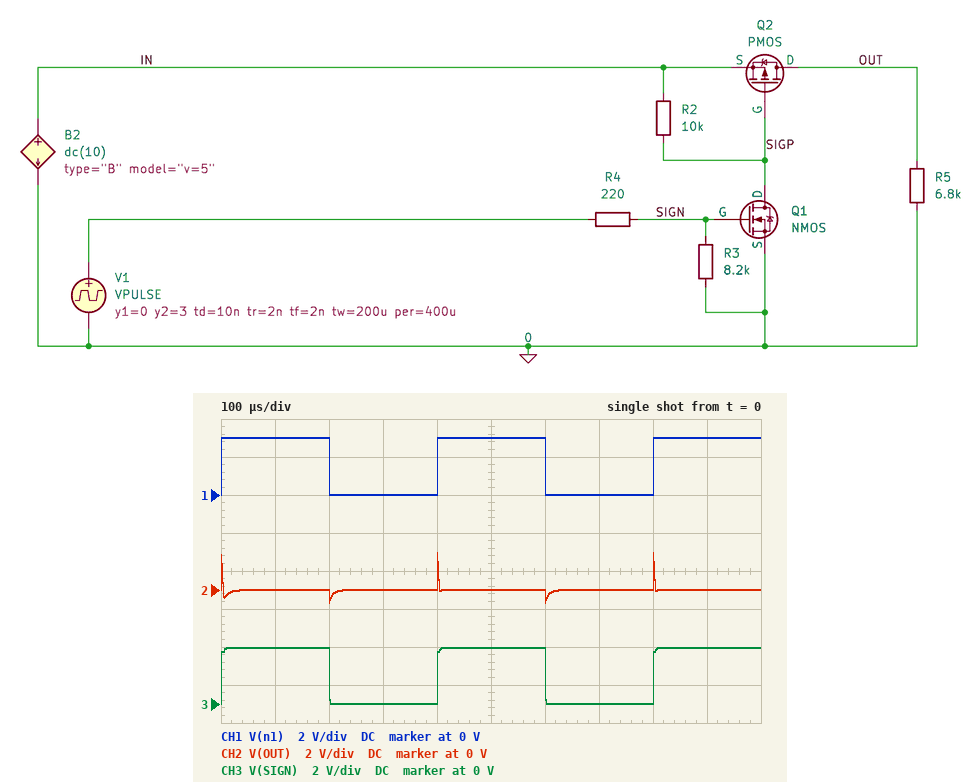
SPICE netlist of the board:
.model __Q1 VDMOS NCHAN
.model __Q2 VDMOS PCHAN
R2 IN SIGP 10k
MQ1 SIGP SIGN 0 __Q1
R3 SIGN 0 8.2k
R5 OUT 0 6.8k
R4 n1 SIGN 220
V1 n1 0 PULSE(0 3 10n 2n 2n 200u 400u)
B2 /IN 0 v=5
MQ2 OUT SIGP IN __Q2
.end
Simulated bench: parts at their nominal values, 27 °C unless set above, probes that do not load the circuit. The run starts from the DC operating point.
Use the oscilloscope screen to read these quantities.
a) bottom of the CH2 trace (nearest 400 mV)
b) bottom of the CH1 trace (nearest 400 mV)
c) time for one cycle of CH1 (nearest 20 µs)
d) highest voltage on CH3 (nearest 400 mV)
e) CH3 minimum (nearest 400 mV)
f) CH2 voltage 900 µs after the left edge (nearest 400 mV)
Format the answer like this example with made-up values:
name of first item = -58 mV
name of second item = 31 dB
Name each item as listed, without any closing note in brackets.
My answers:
bottom of the CH2 trace = -800 mV
bottom of the CH1 trace = 0 V
time for one cycle of CH1 = 400 µs
highest voltage on CH3 = 2.8 V
CH3 minimum = 0 V
CH2 voltage 900 µs after the left edge = 0 V
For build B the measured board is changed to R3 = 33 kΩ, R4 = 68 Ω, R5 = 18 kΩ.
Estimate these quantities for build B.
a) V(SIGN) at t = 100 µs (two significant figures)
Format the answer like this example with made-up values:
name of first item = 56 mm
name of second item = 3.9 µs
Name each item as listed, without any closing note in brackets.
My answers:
V(SIGN) at t = 100 µs = 3.0 V
